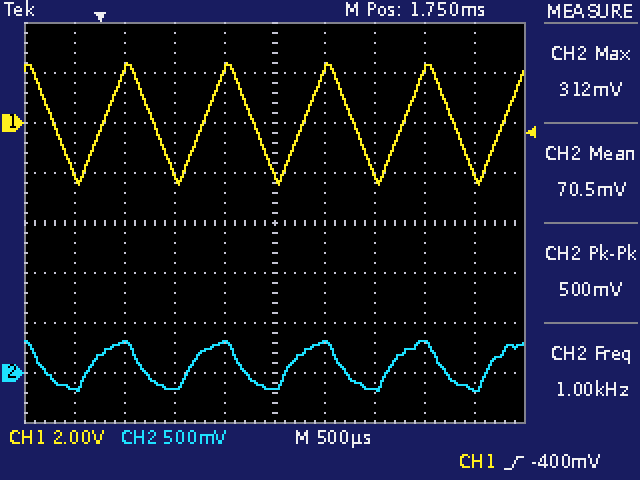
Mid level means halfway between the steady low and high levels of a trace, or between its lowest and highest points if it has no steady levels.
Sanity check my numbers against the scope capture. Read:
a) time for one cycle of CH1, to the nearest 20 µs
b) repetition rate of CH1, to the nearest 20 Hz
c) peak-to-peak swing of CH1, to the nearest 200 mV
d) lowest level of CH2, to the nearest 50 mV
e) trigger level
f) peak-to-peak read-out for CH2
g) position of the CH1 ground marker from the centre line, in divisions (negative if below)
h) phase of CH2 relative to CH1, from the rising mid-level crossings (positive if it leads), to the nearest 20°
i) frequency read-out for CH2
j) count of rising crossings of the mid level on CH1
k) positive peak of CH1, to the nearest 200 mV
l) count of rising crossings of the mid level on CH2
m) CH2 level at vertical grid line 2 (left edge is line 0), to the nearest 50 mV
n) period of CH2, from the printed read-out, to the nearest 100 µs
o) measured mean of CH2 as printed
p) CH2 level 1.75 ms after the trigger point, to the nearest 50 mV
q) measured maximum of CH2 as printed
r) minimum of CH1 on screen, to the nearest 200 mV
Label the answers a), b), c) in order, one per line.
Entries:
a) 1.00 ms
b) 1.00 kHz
c) 4.8 V
d) -200 mV
e) -400 mV
f) 500 mV
g) +2.0 div
h) +40°
i) 1.00 kHz
j) 5
k) 2.4 V
l) 5
m) 300 mV
n) 1.0 ms
o) 70.5 mV
p) -150 mV
q) 312 mV
r) -2.4 V
